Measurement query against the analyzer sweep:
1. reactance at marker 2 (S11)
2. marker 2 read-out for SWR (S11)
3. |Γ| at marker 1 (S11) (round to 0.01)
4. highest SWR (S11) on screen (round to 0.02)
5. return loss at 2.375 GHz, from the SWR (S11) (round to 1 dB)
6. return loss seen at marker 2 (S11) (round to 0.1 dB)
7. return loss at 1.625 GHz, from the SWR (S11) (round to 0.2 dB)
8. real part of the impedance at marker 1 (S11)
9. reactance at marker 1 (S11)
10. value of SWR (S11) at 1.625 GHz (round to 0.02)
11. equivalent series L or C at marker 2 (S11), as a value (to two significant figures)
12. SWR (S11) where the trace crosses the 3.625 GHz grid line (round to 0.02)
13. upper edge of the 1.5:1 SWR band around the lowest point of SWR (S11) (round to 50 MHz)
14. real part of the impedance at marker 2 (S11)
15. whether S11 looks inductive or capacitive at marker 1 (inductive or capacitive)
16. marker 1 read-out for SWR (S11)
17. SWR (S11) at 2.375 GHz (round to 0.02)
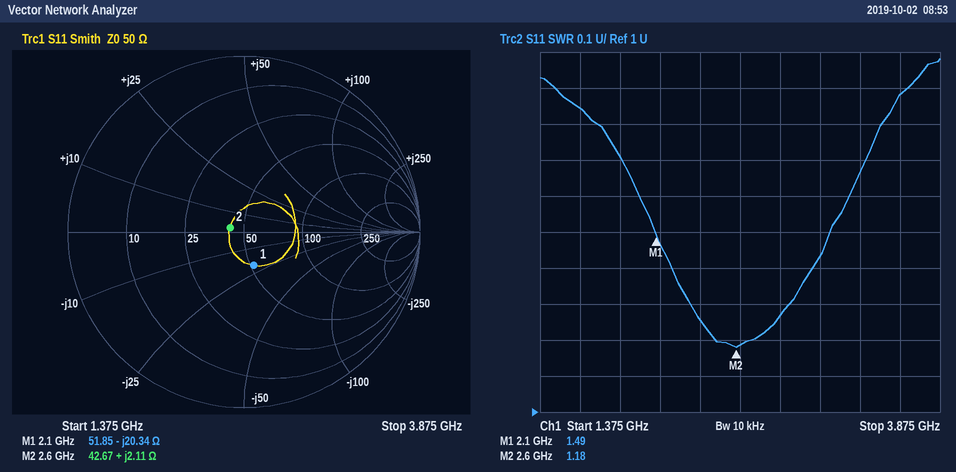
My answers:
+2.11 Ω
1.18
0.20
1.98
19 dB
21.7 dB
10.6 dB
51.85 Ω
-20.34 Ω
1.84
130 pH
1.88
3.20 GHz
42.67 Ω
capacitive
1.49
1.26
